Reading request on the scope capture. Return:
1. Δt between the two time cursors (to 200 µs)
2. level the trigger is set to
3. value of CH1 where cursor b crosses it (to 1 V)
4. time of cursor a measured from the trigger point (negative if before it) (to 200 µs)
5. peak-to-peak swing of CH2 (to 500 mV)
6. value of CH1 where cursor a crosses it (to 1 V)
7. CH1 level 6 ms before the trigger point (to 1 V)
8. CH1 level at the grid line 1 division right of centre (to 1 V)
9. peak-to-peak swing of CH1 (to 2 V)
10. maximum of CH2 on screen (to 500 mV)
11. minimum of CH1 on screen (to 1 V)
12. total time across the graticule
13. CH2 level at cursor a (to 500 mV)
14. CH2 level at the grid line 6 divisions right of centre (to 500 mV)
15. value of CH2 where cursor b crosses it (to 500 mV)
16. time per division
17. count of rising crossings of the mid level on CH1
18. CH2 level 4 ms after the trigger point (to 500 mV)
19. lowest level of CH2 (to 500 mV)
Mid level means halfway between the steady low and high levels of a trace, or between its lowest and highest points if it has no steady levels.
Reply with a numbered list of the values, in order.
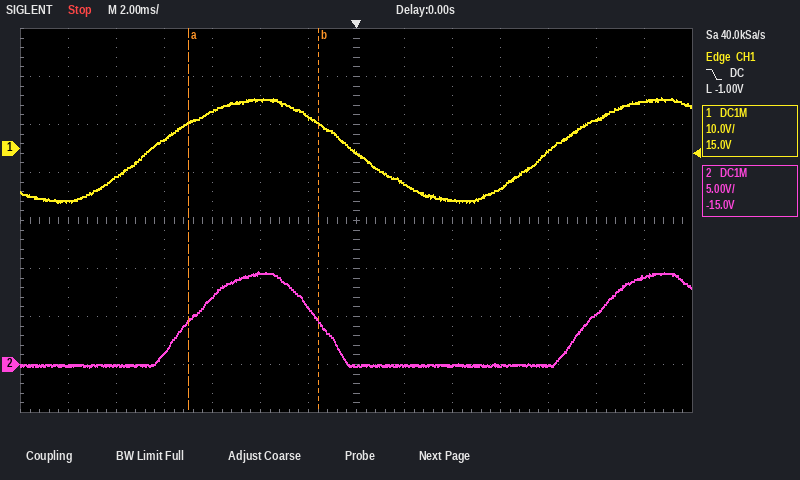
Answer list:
1. 5.4 ms
2. -1.00 V
3. 5 V
4. -7.0 ms
5. 10.0 V
6. 5 V
7. 8 V
8. -7 V
9. 22 V
10. 9.5 V
11. -11 V
12. 28 ms
13. 4.5 V
14. 9.0 V
15. 4.5 V
16. 2 ms
17. 2
18. 0.0 V
19. -500 mV
